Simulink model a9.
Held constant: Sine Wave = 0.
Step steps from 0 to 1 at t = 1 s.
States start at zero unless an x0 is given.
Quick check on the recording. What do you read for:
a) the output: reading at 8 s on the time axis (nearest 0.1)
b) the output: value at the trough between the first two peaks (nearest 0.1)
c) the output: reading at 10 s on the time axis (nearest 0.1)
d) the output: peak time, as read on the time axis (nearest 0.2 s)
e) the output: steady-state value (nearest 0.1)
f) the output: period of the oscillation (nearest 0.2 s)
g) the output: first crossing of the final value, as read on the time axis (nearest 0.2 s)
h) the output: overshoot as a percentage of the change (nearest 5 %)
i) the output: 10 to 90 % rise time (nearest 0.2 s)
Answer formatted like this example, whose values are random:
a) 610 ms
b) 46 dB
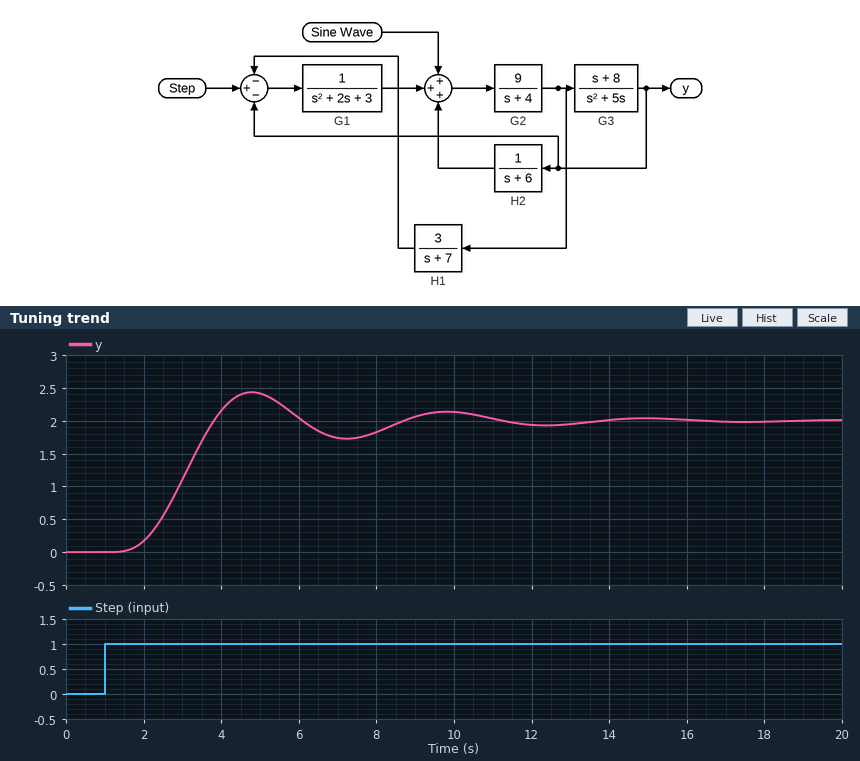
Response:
a) 1.8
b) 1.7
c) 2.1
d) 4.8 s
e) 2.0
f) 5.0 s
g) 3.8 s
h) 20 %
i) 1.6 s
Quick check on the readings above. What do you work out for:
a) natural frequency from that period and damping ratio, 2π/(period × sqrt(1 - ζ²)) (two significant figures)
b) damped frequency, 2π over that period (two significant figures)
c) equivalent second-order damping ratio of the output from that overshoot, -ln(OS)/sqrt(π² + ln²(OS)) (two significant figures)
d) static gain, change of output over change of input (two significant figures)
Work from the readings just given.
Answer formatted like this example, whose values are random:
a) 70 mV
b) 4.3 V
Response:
a) 1.4 rad/s
b) 1.3 rad/s
c) 0.46
d) 2.0
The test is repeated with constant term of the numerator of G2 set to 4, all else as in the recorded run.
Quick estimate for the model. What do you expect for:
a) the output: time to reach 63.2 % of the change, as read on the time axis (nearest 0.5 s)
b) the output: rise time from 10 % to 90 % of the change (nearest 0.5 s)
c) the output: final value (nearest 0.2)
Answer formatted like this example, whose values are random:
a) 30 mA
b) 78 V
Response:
a) 4.5 s
b) 6.0 s
c) 2.0
